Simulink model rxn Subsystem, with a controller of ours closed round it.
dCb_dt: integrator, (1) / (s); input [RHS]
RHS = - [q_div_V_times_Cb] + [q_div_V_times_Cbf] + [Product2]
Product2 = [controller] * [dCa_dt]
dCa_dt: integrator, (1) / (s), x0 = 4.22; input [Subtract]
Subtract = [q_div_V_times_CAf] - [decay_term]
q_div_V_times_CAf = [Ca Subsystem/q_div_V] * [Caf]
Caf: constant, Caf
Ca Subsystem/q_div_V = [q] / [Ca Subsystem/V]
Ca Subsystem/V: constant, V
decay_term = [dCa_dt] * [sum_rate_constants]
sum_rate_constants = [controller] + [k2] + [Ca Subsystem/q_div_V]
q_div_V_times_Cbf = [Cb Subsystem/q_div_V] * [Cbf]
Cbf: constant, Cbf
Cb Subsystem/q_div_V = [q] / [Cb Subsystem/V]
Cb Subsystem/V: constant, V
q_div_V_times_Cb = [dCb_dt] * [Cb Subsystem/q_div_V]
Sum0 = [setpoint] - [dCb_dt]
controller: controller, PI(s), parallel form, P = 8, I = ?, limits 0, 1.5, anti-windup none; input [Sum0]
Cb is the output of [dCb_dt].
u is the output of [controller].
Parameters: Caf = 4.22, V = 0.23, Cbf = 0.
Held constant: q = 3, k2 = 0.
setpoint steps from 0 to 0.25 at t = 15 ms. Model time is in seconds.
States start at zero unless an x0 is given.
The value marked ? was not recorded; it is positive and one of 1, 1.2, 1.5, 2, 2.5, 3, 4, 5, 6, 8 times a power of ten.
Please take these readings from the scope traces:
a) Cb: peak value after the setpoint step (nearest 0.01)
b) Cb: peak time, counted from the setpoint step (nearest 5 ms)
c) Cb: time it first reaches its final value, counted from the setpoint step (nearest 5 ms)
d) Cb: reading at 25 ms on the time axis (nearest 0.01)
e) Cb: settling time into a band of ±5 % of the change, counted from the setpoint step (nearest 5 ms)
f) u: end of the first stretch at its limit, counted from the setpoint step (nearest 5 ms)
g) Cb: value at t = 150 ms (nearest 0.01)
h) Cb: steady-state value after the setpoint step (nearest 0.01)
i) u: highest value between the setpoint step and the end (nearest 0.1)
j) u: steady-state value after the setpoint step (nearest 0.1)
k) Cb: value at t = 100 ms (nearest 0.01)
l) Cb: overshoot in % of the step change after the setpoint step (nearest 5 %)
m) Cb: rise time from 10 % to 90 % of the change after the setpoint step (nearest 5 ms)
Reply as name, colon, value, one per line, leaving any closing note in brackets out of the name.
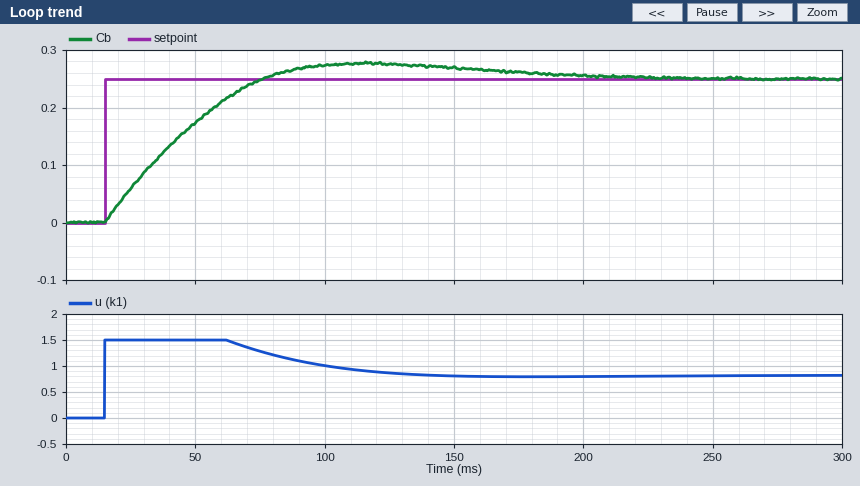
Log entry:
Cb: peak value after the setpoint step: 0.28
Cb: peak time, counted from the setpoint step: 100 ms
Cb: time it first reaches its final value, counted from the setpoint step: 60 ms
Cb: reading at 25 ms on the time axis: 0.06
Cb: settling time into a band of ±5 % of the change, counted from the setpoint step: 155 ms
u: end of the first stretch at its limit, counted from the setpoint step: 50 ms
Cb: value at t = 150 ms: 0.27
Cb: steady-state value after the setpoint step: 0.25
u: highest value between the setpoint step and the end: 1.5
u: steady-state value after the setpoint step: 0.8
Cb: value at t = 100 ms: 0.27
Cb: overshoot in % of the step change after the setpoint step: 10 %
Cb: rise time from 10 % to 90 % of the change after the setpoint step: 45 ms
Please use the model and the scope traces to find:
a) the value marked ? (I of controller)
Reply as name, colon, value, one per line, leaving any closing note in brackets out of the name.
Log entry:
the value marked ?: 200
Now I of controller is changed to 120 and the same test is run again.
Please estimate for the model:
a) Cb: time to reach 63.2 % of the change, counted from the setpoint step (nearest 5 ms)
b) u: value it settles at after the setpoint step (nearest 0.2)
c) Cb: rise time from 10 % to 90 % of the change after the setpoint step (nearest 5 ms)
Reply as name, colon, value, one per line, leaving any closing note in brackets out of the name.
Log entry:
Cb: time to reach 63.2 % of the change, counted from the setpoint step: 30 ms
u: value it settles at after the setpoint step: 0.8
Cb: rise time from 10 % to 90 % of the change after the setpoint step: 60 ms
